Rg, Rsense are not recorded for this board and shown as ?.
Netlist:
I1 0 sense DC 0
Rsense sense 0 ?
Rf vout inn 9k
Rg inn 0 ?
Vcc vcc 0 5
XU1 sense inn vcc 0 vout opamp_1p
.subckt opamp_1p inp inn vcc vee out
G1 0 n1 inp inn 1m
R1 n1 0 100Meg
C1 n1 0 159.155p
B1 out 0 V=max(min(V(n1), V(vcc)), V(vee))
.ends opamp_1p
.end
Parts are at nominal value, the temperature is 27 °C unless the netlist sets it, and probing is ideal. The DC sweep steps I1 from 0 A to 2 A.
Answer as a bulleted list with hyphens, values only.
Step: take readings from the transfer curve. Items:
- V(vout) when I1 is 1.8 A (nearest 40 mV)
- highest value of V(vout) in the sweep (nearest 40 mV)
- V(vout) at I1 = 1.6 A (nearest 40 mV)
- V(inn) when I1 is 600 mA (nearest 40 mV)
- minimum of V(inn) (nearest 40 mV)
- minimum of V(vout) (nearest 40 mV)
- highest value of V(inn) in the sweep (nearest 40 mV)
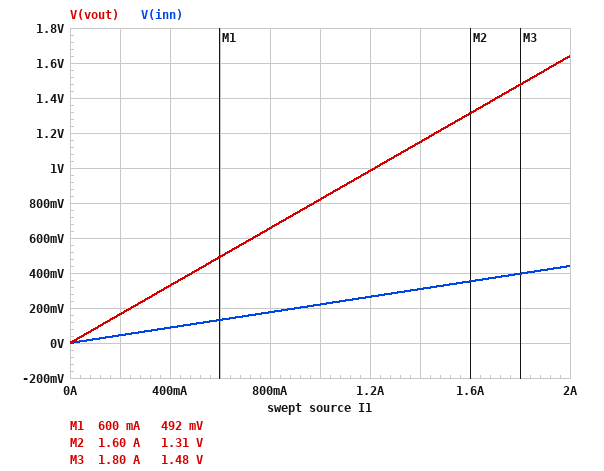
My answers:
- 1.48 V
- 1.64 V
- 1.32 V
- 120 mV
- 0 V
- 0 V
- 440 mV
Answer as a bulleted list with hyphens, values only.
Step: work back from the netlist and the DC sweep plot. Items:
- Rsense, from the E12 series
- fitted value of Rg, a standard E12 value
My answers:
- 0.22 Ω
- 3.3 kΩ
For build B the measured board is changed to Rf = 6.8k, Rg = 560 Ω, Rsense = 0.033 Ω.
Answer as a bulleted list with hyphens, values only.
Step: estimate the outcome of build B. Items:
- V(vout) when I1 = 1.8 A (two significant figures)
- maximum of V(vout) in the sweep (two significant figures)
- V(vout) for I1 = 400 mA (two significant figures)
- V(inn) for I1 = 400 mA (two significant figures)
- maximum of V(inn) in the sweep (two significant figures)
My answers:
- 780 mV
- 870 mV
- 170 mV
- 13 mV
- 66 mV
